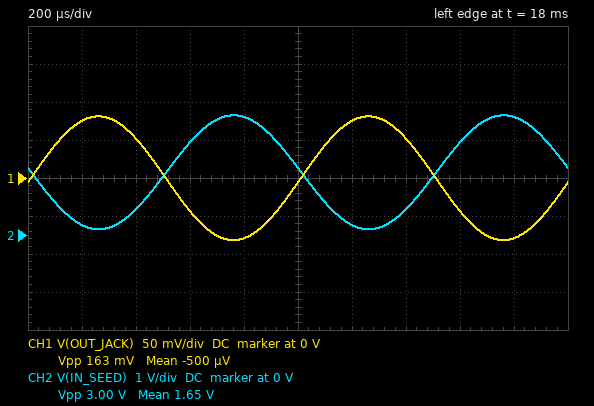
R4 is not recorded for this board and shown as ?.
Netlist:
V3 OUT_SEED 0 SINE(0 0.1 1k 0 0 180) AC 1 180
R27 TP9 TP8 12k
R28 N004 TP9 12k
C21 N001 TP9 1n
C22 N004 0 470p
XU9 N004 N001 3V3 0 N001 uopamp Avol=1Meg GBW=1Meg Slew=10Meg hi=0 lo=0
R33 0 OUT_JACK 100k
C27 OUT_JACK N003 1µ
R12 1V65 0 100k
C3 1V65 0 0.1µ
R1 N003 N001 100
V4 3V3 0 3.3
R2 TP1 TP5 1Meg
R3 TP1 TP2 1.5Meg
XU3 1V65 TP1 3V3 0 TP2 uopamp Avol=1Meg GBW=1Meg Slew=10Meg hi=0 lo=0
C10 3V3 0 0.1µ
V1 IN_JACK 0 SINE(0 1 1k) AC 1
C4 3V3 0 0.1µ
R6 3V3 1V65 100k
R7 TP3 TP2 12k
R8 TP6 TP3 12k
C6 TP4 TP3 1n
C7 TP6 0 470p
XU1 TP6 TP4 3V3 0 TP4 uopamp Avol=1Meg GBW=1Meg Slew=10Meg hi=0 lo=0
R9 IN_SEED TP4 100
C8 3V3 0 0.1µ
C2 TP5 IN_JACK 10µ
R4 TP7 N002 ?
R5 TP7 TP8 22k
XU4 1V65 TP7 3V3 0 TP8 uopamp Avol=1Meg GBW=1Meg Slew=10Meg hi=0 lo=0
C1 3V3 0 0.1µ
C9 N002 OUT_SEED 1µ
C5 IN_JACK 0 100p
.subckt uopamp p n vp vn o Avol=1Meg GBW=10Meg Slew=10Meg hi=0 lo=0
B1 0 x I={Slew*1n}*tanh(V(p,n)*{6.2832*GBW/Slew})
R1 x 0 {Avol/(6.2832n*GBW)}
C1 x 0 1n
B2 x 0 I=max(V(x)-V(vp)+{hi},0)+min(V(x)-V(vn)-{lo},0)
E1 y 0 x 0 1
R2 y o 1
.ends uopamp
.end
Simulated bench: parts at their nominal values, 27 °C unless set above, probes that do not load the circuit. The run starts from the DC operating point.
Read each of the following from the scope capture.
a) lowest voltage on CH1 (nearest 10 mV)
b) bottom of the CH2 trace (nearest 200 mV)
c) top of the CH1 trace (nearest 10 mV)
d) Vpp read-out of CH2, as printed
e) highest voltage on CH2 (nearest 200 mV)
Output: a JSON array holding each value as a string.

["-80 mV", "200 mV", "80 mV", "3.00 V", "3.2 V"]
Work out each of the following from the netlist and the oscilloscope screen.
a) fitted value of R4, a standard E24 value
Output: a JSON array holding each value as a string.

["27 kΩ"]
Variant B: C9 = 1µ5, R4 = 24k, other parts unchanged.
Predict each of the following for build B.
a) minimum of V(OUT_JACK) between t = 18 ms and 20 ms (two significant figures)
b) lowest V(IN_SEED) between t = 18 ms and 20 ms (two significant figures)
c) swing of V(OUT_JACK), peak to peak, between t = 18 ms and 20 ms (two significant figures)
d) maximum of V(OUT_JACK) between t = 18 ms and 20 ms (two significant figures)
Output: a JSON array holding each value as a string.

["-92 mV", "150 mV", "180 mV", "91 mV"]
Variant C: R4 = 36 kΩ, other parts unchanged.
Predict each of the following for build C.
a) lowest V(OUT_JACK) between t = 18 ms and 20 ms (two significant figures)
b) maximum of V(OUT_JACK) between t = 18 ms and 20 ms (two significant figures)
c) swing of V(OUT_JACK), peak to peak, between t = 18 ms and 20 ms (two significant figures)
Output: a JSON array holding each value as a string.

["-61 mV", "61 mV", "120 mV"]
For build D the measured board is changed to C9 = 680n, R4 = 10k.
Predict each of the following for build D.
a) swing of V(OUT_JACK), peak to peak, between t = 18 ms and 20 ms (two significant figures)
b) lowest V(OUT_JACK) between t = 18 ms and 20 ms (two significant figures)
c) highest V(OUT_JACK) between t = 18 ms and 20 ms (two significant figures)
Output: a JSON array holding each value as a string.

["440 mV", "-220 mV", "220 mV"]
